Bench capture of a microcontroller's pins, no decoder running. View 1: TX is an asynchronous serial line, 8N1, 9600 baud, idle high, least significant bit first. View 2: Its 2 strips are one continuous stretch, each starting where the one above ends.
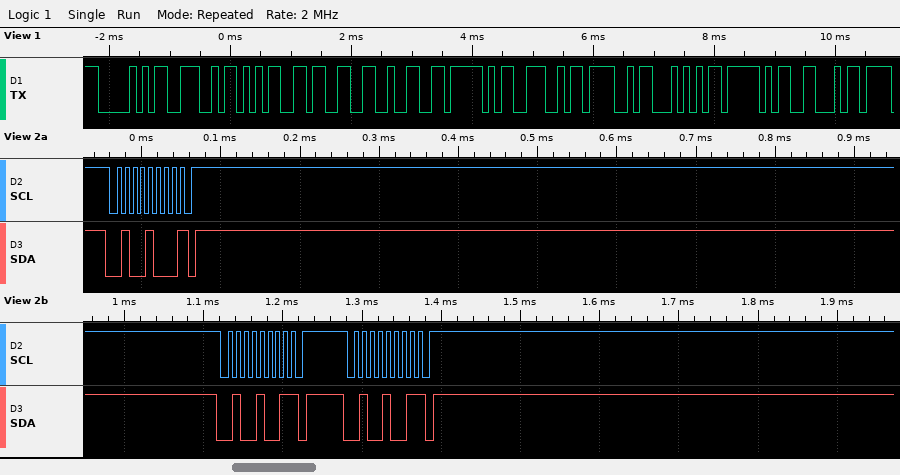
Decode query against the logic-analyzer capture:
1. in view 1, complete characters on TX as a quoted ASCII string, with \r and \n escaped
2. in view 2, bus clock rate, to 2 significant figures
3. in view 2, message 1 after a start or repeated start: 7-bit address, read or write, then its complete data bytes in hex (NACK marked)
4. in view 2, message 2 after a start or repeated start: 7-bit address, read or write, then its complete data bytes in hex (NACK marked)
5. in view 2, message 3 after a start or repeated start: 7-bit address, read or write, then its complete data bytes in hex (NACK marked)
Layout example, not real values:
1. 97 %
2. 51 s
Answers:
1. "PN532_NOT_F"
2. 100 kHz
3. 0x24 write NACK
4. 0x24 read NACK
5. 0x24 read NACK
